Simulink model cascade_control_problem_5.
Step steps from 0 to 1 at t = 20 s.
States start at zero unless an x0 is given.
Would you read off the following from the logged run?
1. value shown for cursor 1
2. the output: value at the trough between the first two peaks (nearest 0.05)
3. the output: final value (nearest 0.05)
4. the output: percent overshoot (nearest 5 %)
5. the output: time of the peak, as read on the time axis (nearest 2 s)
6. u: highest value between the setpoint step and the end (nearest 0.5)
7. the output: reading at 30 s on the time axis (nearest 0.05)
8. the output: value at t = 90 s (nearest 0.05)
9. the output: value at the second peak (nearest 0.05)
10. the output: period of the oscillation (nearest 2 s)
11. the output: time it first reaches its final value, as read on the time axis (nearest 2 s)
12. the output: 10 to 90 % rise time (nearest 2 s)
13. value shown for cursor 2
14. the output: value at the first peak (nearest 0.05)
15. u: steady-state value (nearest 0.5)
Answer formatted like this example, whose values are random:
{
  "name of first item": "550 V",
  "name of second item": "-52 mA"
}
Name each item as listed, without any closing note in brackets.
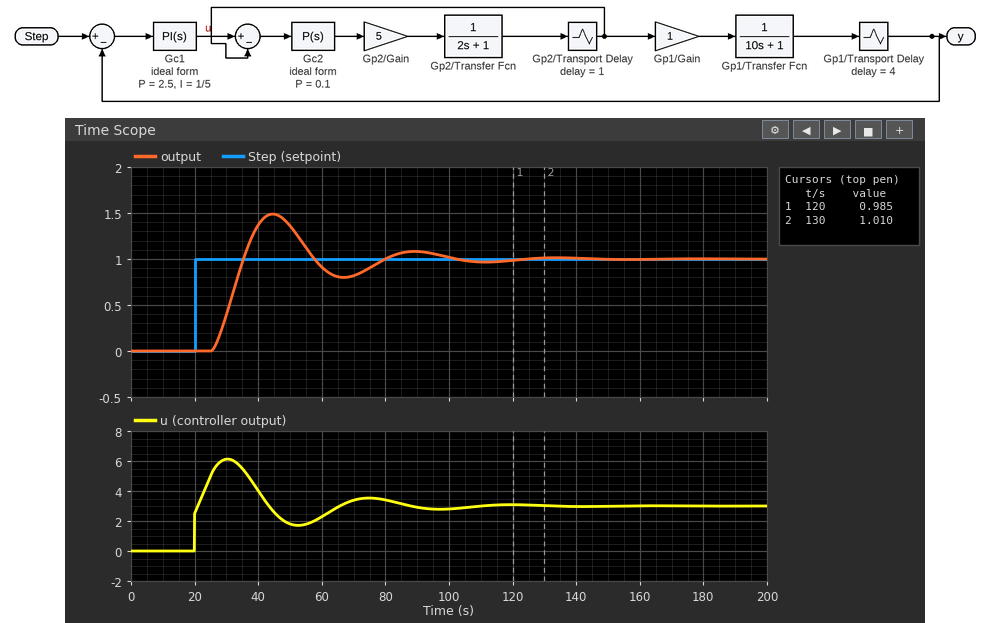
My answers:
{
  "value shown for cursor 1": "0.985",
  "the output: value at the trough between the first two peaks": "0.80",
  "the output: final value": "1.00",
  "the output: percent overshoot": "50 %",
  "the output: time of the peak, as read on the time axis": "44 s",
  "u: highest value between the setpoint step and the end": "6.0",
  "the output: reading at 30 s on the time axis": "0.40",
  "the output: value at t = 90 s": "1.10",
  "the output: value at the second peak": "1.10",
  "the output: period of the oscillation": "44 s",
  "the output: time it first reaches its final value, as read on the time axis": "36 s",
  "the output: 10 to 90 % rise time": "8 s",
  "value shown for cursor 2": "1.010",
  "the output: value at the first peak": "1.50",
  "u: steady-state value": "3.0"
}
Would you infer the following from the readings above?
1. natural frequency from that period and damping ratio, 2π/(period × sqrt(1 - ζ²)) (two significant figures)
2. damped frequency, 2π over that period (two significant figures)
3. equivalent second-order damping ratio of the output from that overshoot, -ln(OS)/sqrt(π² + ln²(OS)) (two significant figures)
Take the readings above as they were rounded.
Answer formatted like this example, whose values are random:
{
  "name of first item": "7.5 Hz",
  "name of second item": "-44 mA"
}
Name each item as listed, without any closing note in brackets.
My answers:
{
  "natural frequency from that period and damping ratio, 2π/(period × sqrt(1 - ζ²))": "0.15 rad/s",
  "damped frequency, 2π over that period": "0.14 rad/s",
  "equivalent second-order damping ratio of the output from that overshoot, -ln(OS)/sqrt(π² + ln²(OS))": "0.22"
}
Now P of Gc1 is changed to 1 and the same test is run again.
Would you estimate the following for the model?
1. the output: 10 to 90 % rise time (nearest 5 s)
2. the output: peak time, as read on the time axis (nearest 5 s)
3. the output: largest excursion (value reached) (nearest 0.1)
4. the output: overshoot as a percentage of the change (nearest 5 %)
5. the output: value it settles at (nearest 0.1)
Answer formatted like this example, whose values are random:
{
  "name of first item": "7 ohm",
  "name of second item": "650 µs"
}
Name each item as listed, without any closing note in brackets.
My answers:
{
  "the output: 10 to 90 % rise time": "20 s",
  "the output: peak time, as read on the time axis": "65 s",
  "the output: largest excursion (value reached)": "1.1",
  "the output: overshoot as a percentage of the change": "10 %",
  "the output: value it settles at": "1.0"
}
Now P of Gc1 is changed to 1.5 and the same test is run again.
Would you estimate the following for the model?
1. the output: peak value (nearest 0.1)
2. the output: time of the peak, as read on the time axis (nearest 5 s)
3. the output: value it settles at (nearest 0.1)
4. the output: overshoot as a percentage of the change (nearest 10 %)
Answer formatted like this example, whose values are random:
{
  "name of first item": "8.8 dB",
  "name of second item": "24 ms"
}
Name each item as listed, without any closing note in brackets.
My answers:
{
  "the output: peak value": "1.2",
  "the output: time of the peak, as read on the time axis": "55 s",
  "the output: value it settles at": "1.0",
  "the output: overshoot as a percentage of the change": "20 %"
}
